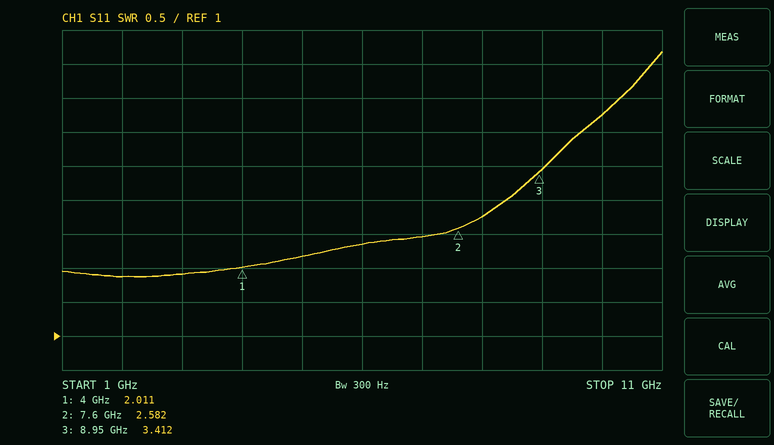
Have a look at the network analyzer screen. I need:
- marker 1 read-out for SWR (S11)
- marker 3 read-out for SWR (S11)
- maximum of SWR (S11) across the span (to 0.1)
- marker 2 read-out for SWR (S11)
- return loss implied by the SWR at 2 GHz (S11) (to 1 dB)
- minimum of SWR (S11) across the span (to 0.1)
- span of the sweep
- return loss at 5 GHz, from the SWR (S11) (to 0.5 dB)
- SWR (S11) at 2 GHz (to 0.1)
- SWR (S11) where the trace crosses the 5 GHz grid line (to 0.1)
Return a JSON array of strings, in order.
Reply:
["2.011", "3.412", "5.2", "2.582", "10 dB", "1.9", "10 GHz", "8.5 dB", "1.9", "2.2"]
